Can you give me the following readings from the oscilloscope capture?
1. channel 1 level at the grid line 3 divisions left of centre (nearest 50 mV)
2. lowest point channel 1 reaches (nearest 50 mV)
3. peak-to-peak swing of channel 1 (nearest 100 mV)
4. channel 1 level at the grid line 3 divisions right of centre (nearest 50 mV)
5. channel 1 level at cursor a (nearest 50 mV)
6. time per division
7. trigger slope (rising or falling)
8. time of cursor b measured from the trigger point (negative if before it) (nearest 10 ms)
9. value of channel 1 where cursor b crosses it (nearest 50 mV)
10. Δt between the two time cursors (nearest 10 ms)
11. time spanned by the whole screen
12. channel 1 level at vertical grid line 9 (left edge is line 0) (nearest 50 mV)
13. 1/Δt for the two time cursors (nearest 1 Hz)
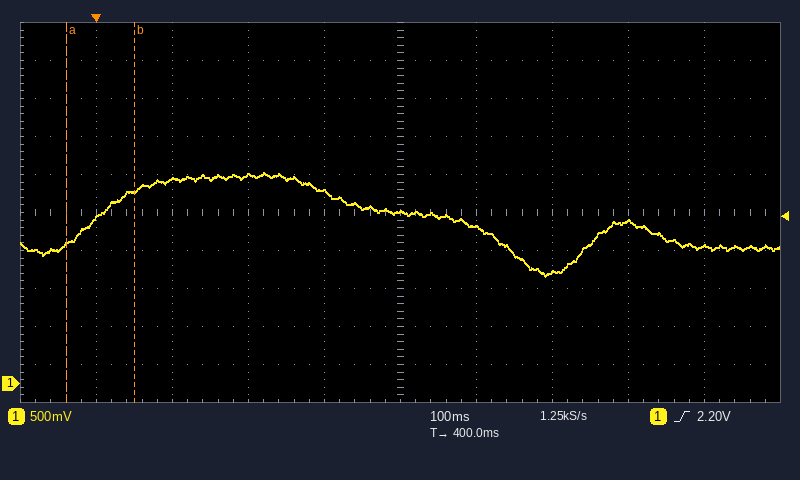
2.70 V
1.40 V
1.40 V
2.15 V
1.85 V
100 ms
rising
+50 ms
2.55 V
90 ms
1 s
1.80 V
11 Hz
